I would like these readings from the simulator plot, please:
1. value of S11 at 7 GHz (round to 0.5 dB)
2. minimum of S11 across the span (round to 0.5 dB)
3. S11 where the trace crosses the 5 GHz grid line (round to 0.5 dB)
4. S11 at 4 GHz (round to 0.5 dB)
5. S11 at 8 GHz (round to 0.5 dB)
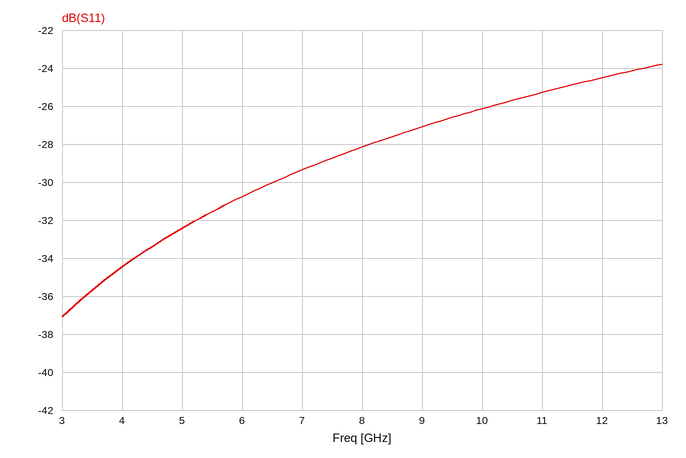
-29.5 dB
-37.0 dB
-32.5 dB
-34.5 dB
-28.0 dB
